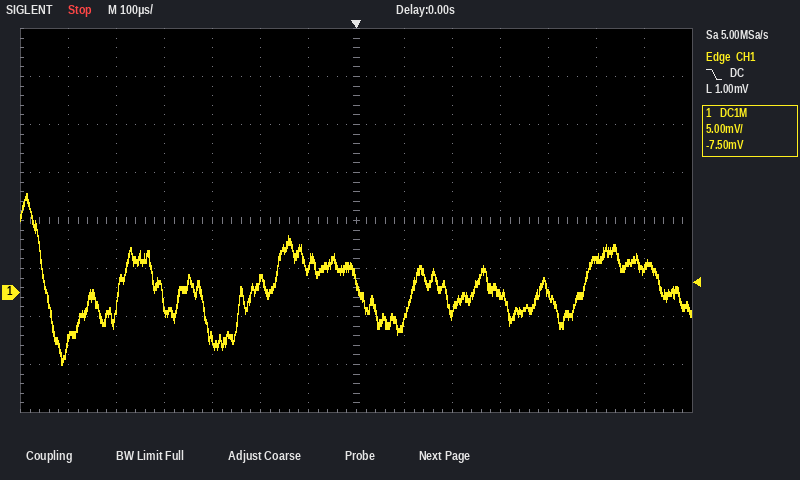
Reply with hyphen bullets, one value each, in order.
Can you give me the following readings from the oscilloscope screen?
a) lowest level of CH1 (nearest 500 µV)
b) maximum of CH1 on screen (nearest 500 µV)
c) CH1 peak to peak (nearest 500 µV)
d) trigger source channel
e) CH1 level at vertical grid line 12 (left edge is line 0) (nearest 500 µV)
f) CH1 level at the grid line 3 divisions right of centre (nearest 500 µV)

- -7.5 mV
- 10.5 mV
- 18.0 mV
- CH1
- 3.5 mV
- 0.0 mV
